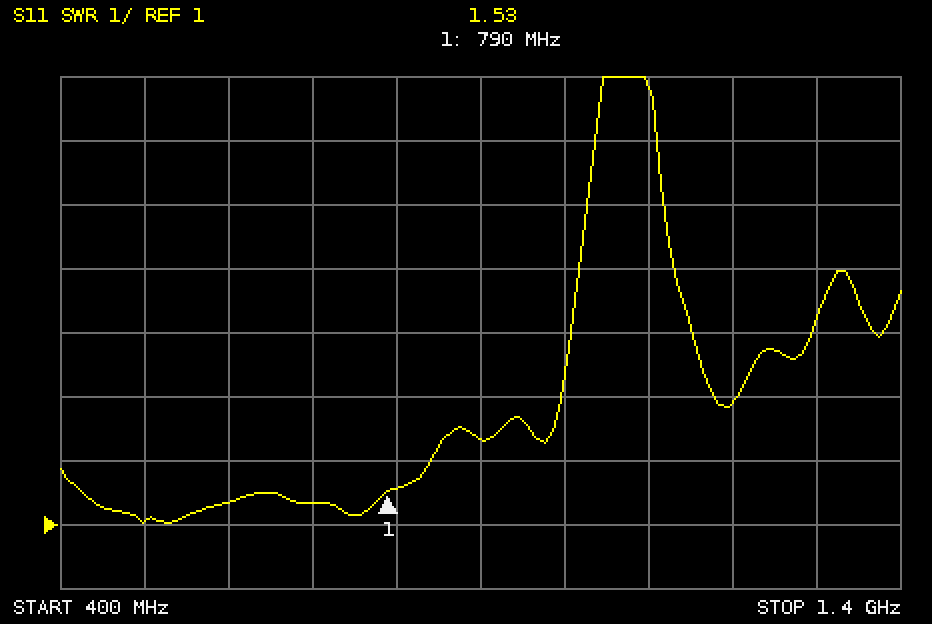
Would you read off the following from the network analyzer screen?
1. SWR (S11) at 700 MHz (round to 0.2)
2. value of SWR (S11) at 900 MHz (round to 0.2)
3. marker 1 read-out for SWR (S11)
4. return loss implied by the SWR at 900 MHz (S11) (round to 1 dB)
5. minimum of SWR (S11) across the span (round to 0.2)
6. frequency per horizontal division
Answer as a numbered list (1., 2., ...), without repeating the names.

1. 1.4
2. 2.4
3. 1.53
4. 8 dB
5. 1.0
6. 100 MHz
